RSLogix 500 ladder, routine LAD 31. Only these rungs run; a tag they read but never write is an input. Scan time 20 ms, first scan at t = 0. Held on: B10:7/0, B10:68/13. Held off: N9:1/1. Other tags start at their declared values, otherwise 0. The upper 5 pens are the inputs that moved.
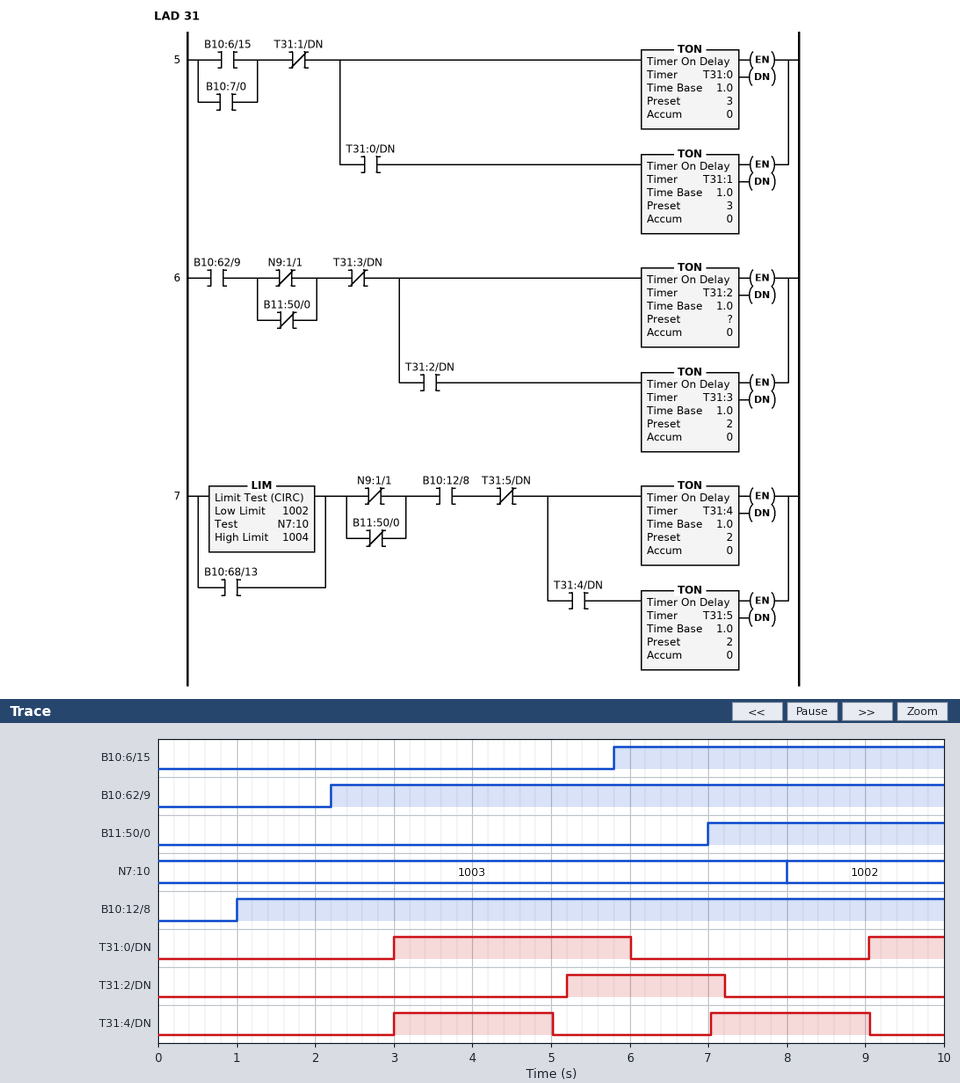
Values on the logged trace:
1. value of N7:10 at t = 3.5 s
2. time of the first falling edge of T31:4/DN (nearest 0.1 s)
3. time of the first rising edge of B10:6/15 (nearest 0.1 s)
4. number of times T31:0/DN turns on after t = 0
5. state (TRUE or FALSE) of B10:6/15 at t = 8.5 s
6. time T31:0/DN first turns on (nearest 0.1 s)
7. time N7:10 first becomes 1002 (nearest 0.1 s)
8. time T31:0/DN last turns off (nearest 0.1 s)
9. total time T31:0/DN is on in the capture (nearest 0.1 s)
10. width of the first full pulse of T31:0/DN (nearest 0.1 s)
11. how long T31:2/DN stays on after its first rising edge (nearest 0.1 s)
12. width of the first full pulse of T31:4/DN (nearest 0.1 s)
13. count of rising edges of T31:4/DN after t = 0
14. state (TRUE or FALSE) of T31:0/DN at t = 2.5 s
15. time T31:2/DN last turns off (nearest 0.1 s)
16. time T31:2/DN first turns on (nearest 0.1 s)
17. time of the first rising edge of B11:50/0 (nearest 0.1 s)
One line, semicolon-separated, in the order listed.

1003; 5.0 s; 5.8 s; 2; TRUE; 3.0 s; 8.0 s; 6.0 s; 4.0 s; 3.0 s; 2.0 s; 2.0 s; 2; FALSE; 7.2 s; 5.2 s; 7.0 s
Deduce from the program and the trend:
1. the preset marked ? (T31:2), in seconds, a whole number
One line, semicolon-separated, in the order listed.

3 s
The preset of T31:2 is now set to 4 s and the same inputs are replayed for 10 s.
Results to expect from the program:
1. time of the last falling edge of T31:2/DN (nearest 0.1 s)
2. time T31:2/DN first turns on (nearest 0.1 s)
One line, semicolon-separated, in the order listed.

8.2 s; 6.2 s
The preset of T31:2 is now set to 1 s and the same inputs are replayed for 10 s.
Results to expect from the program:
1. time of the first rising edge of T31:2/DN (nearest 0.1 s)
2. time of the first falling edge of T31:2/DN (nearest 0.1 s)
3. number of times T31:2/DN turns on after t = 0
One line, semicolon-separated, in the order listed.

3.2 s; 5.2 s; 3
